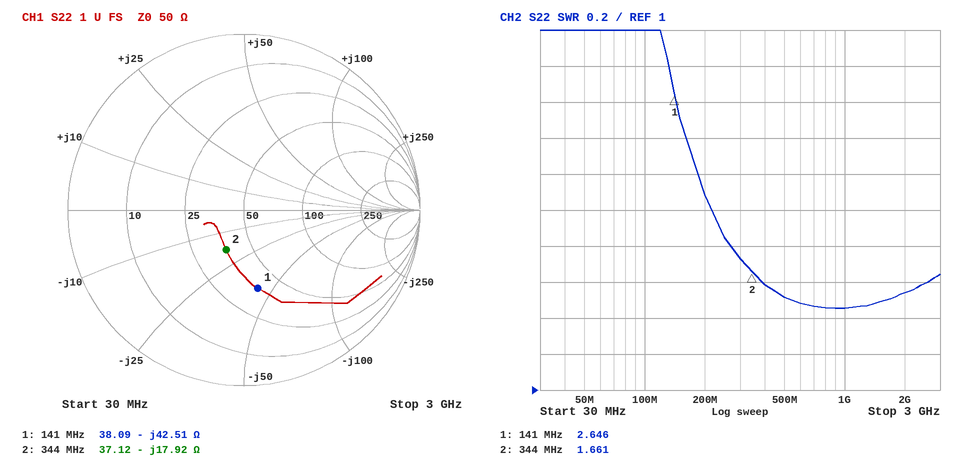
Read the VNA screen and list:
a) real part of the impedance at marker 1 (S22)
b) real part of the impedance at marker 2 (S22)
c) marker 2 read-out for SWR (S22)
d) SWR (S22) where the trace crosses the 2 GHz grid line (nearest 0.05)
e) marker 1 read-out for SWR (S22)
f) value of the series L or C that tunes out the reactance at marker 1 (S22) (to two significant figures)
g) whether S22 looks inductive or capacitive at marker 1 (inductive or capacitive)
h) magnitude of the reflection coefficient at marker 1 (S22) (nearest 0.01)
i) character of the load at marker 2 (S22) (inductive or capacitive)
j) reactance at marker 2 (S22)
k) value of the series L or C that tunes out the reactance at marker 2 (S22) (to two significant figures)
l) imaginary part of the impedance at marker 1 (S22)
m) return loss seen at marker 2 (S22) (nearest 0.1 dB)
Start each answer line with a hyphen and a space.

- 38.09 Ω
- 37.12 Ω
- 1.661
- 1.55
- 2.646
- 48 nH
- capacitive
- 0.45
- capacitive
- -17.92 Ω
- 8.3 nH
- -42.51 Ω
- 12.1 dB
